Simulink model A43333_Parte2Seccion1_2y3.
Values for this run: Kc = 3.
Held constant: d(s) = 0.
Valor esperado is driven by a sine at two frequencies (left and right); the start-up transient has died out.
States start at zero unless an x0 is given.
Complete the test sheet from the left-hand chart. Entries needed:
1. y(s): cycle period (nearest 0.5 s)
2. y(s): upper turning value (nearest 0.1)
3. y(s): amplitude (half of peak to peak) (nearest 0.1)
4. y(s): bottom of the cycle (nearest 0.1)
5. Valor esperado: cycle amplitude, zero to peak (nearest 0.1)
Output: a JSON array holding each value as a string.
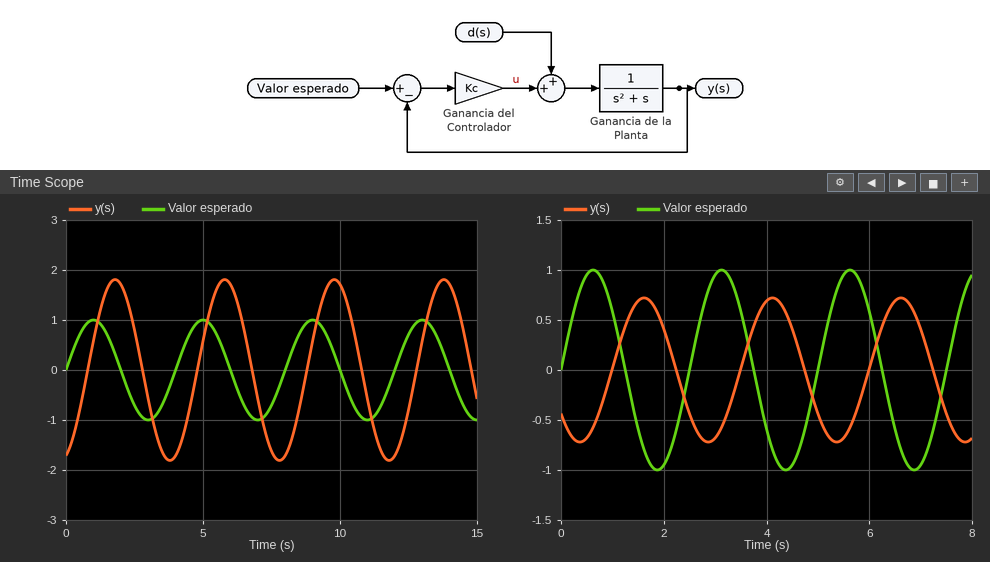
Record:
["4.0 s", "1.8", "1.8", "-1.8", "1.0"]
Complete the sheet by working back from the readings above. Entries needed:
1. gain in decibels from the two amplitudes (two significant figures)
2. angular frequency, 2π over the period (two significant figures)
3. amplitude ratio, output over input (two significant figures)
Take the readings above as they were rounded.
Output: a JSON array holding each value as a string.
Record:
["5.1 dB", "1.6 rad/s", "1.8"]
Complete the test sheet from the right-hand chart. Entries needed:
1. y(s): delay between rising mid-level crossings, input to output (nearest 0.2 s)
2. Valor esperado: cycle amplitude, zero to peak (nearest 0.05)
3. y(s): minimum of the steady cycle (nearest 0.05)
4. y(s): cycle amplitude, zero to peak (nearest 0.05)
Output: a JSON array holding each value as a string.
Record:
["1.0 s", "1.00", "-0.70", "0.70"]
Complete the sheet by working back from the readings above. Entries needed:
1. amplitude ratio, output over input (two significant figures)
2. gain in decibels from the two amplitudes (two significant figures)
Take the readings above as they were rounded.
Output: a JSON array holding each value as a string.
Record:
["0.70", "-3.1 dB"]
